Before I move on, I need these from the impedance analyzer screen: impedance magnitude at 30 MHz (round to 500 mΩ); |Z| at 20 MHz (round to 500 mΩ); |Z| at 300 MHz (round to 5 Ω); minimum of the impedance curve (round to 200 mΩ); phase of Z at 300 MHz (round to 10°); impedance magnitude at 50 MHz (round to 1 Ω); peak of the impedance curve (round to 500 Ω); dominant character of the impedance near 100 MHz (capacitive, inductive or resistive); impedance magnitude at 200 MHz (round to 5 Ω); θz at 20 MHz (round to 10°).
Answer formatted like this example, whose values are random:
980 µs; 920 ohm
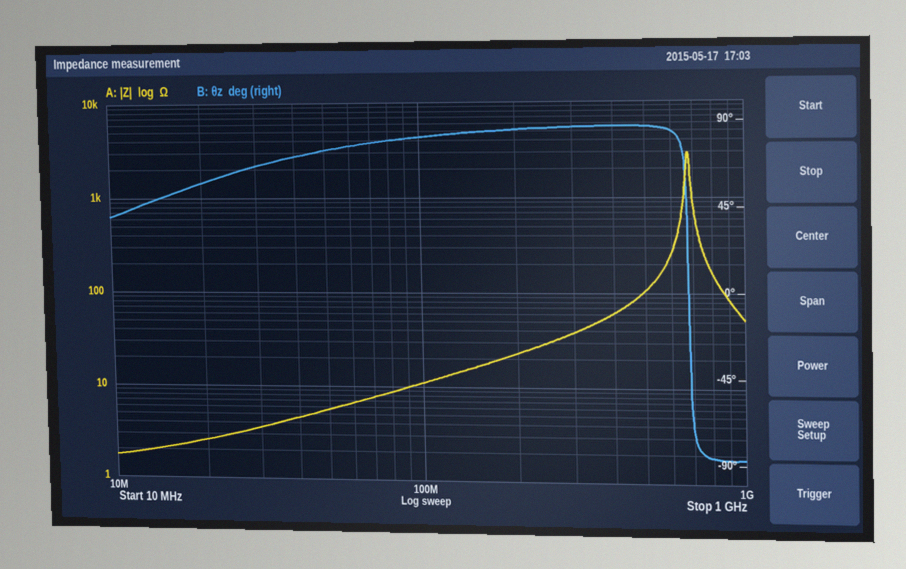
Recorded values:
3.5 Ω; 2.5 Ω; 40 Ω; 1.8 Ω; 90°; 6 Ω; 3.0 kΩ; inductive; 25 Ω; 60°
